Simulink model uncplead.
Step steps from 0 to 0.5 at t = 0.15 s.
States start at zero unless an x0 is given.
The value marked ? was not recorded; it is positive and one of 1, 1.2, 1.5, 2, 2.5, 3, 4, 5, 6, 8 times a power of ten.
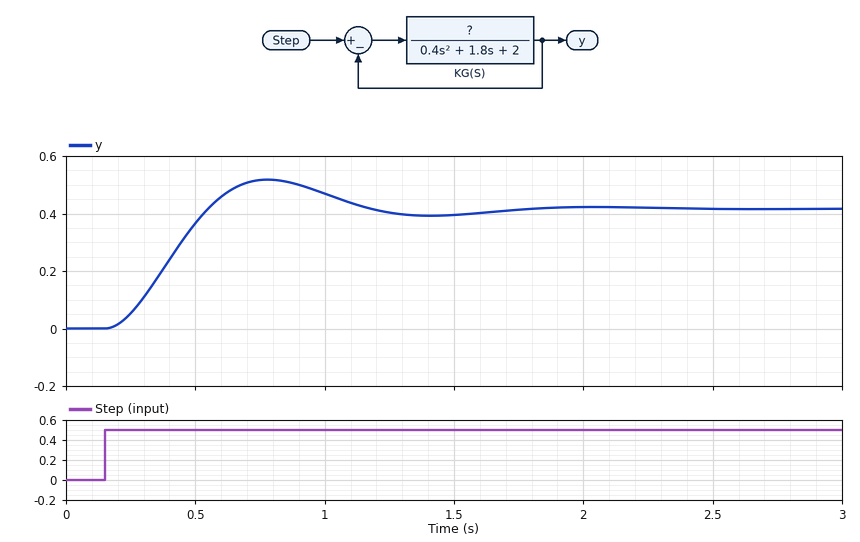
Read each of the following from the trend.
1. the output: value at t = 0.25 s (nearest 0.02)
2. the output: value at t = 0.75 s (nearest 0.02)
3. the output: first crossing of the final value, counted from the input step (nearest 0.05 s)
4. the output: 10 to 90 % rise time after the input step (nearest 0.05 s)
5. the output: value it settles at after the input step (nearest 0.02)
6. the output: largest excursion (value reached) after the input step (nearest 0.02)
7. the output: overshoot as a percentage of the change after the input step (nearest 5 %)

0.06
0.52
0.40 s
0.25 s
0.42
0.52
25 %
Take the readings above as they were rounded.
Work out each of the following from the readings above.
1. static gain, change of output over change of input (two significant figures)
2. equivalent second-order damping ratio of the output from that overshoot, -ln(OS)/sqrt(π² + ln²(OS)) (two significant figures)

0.84
0.40
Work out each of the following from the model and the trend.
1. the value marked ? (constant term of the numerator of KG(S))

10
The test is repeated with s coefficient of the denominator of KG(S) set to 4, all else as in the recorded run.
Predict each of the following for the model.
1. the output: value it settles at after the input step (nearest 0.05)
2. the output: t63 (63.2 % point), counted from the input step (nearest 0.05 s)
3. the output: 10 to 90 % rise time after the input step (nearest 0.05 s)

0.40
0.35 s
0.55 s
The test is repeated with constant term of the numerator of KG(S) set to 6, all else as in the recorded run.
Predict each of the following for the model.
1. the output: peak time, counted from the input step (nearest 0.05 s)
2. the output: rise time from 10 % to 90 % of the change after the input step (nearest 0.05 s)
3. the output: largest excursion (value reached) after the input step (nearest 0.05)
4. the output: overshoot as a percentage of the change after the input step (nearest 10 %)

0.80 s
0.35 s
0.45
20 %
